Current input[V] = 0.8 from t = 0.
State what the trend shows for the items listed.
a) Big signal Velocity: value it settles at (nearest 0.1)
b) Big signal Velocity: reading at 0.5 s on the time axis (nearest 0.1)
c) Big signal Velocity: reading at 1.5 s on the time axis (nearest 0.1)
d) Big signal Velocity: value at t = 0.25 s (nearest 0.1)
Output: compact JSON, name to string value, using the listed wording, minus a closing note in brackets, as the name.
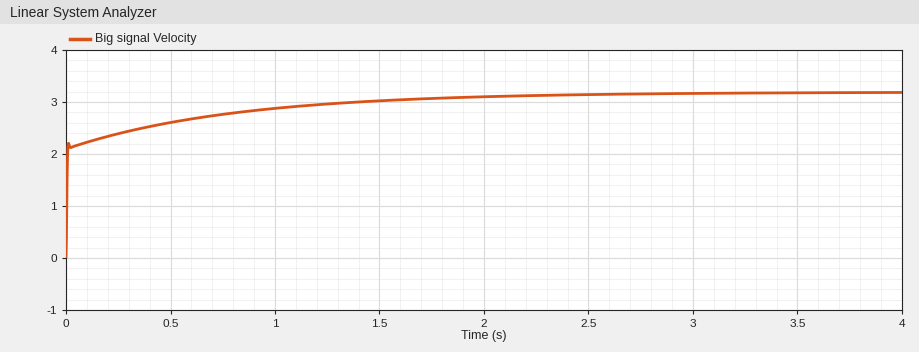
{"Big signal Velocity: value it settles at": "3.2", "Big signal Velocity: reading at 0.5 s on the time axis": "2.6", "Big signal Velocity: reading at 1.5 s on the time axis": "3.0", "Big signal Velocity: value at t = 0.25 s": "2.4"}
